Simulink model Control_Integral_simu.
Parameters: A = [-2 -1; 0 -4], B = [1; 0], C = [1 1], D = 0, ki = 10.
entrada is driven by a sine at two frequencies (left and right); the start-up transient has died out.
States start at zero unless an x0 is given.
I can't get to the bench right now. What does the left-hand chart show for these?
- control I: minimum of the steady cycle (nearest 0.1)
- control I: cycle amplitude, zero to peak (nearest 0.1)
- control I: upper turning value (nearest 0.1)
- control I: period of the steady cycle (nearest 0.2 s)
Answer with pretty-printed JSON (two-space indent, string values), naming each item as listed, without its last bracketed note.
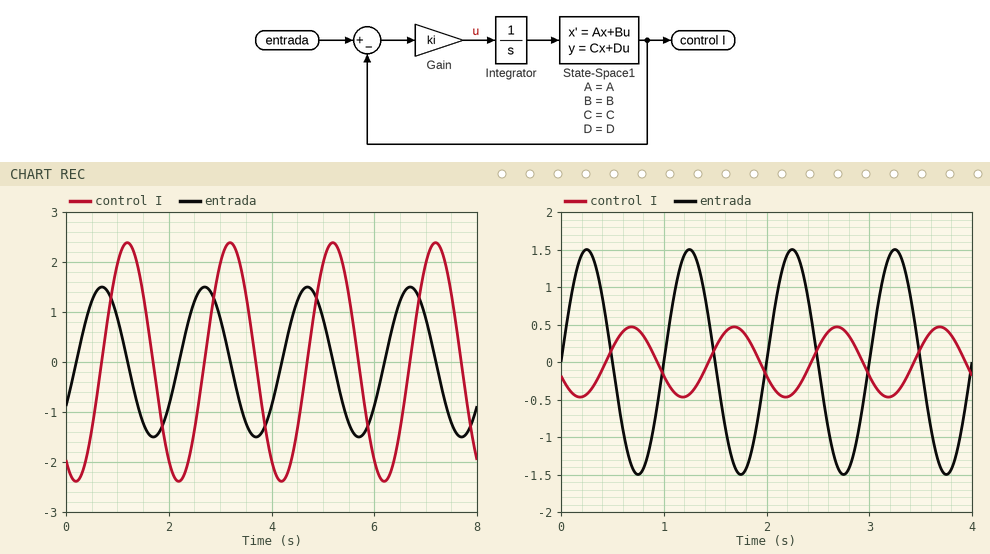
{
  "control I: minimum of the steady cycle": "-2.4",
  "control I: cycle amplitude, zero to peak": "2.4",
  "control I: upper turning value": "2.4",
  "control I: period of the steady cycle": "2.0 s"
}
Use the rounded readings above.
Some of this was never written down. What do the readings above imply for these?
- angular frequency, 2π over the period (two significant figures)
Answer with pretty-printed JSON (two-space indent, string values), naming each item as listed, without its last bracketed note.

{
  "angular frequency, 2π over the period": "3.1 rad/s"
}
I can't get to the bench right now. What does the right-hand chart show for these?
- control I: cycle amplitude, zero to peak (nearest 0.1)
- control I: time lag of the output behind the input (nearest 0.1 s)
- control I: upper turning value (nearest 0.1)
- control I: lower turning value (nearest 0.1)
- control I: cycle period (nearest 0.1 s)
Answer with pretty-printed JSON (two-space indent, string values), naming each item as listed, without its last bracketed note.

{
  "control I: cycle amplitude, zero to peak": "0.5",
  "control I: time lag of the output behind the input": "0.4 s",
  "control I: upper turning value": "0.5",
  "control I: lower turning value": "-0.5",
  "control I: cycle period": "1.0 s"
}
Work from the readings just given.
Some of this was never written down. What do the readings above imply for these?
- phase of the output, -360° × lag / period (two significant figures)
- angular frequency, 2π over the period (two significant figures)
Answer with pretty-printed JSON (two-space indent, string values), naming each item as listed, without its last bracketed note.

{
  "phase of the output, -360° × lag / period": "-140°",
  "angular frequency, 2π over the period": "6.3 rad/s"
}
